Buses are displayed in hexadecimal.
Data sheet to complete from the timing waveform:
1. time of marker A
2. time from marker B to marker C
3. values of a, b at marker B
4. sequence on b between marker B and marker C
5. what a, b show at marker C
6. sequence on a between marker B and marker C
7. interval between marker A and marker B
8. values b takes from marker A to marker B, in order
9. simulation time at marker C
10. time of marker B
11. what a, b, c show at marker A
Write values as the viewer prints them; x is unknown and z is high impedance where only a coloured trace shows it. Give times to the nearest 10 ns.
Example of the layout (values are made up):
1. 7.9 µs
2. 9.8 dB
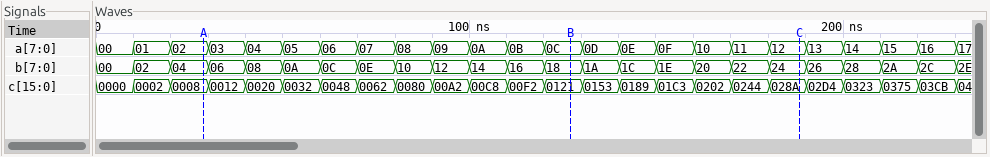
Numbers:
1. 30 ns
2. 60 ns
3. a=0C, b=18
4. 18, 1A, 1C, 1E, 20, 22, 24
5. a=12, b=24
6. 0C, 0D, 0E, 0F, 10, 11, 12
7. 100 ns
8. 04, 06, 08, 0A, 0C, 0E, 10, 12, 14, 16, 18
9. 190 ns
10. 130 ns
11. a=02, b=04, c=0008
